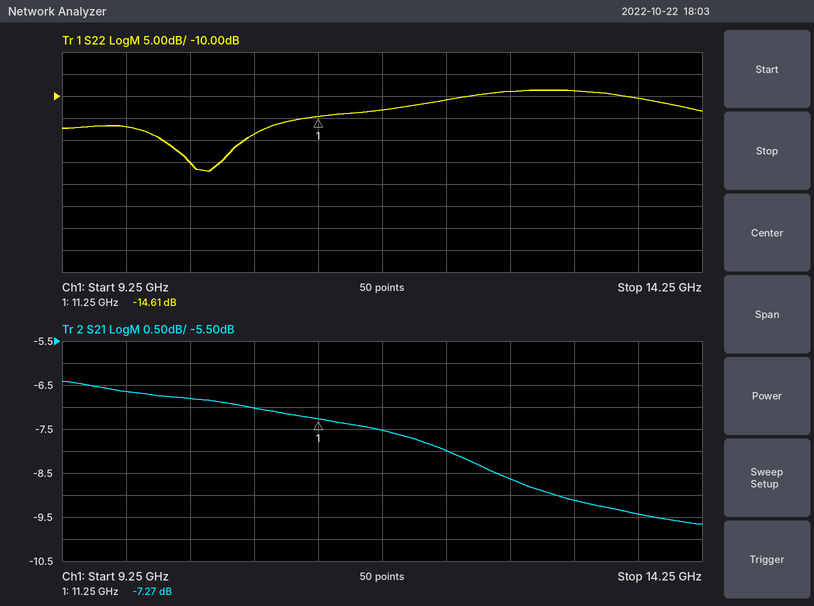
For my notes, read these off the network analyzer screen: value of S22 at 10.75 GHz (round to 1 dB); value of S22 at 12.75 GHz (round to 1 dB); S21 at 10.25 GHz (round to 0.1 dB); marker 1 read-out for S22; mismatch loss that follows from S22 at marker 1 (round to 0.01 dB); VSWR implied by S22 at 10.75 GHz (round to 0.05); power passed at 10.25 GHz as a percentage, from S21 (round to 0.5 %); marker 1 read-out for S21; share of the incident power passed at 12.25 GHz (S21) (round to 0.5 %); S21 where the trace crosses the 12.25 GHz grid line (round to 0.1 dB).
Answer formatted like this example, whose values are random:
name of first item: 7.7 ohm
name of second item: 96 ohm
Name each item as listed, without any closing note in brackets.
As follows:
value of S22 at 10.75 GHz: -19 dB
value of S22 at 12.75 GHz: -9 dB
S21 at 10.25 GHz: -6.8 dB
marker 1 read-out for S22: -14.61 dB
mismatch loss that follows from S22 at marker 1: 0.15 dB
VSWR implied by S22 at 10.75 GHz: 1.25
power passed at 10.25 GHz as a percentage, from S21: 21.0 %
marker 1 read-out for S21: -7.27 dB
share of the incident power passed at 12.25 GHz (S21): 16.0 %
S21 where the trace crosses the 12.25 GHz grid line: -8.0 dB
